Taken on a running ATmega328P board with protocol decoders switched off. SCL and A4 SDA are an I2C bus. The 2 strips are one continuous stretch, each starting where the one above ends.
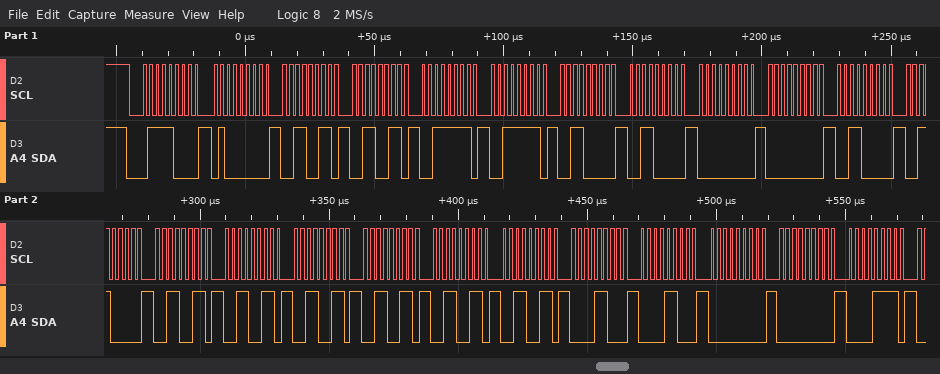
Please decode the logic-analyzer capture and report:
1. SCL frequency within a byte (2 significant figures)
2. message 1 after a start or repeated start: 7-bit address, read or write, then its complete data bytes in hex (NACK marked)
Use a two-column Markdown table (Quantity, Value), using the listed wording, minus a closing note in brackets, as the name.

| Quantity | Value |
|---|---|
| SCL frequency within a byte | 400 kHz |
| message 1 after a start or repeated start: 7-bit address, read or write, then its complete data bytes in hex | 0x3C write: 40 33 33 3F 3F 30 30 00 00 30 30 33 33 33 33 33 33 0C 0C 00 00 0F |
